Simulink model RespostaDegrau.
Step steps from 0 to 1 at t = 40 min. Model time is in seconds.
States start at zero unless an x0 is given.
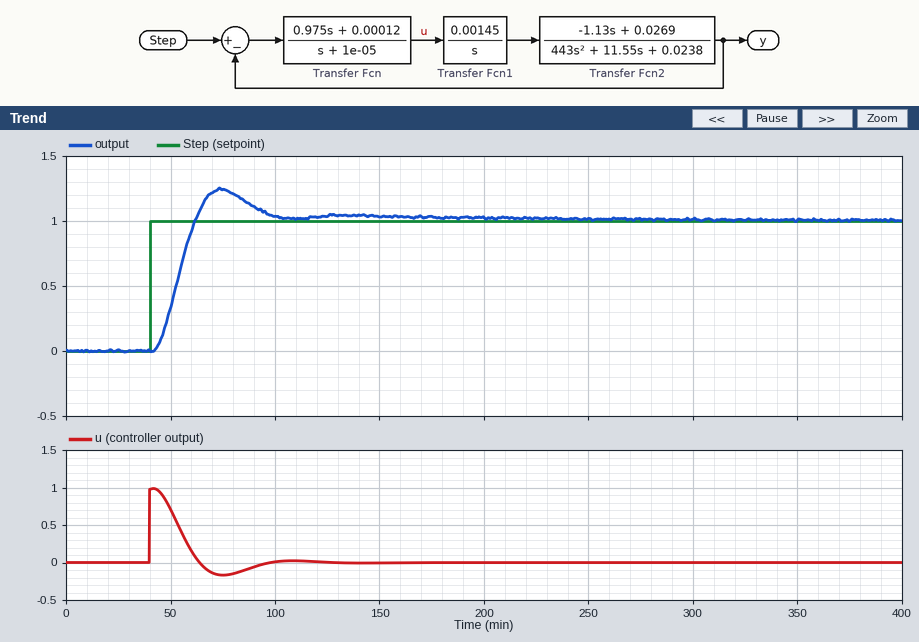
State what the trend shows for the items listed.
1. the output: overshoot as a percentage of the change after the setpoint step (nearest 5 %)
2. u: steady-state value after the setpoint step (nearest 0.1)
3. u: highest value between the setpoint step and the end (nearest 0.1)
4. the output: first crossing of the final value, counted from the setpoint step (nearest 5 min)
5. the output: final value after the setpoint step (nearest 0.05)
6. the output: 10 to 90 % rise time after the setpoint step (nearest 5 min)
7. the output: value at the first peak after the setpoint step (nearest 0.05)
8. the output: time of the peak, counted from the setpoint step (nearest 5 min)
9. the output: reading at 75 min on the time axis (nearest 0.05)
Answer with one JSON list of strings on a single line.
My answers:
["25 %", "0.0", "1.0", "20 min", "1.00", "15 min", "1.25", "35 min", "1.25"]
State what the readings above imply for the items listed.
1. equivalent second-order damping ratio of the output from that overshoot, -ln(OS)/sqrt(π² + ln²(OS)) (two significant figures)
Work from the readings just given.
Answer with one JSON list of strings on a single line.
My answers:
["0.40"]
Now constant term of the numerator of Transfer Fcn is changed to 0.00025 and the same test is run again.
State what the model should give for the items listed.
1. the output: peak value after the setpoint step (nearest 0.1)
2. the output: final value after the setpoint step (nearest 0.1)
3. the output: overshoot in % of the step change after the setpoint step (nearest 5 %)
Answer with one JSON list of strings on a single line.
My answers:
["1.3", "1.0", "35 %"]
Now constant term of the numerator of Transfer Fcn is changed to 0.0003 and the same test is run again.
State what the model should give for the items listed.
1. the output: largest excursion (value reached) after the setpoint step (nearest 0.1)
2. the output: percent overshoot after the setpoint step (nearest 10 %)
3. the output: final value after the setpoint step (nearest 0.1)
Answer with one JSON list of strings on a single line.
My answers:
["1.4", "40 %", "1.0"]
